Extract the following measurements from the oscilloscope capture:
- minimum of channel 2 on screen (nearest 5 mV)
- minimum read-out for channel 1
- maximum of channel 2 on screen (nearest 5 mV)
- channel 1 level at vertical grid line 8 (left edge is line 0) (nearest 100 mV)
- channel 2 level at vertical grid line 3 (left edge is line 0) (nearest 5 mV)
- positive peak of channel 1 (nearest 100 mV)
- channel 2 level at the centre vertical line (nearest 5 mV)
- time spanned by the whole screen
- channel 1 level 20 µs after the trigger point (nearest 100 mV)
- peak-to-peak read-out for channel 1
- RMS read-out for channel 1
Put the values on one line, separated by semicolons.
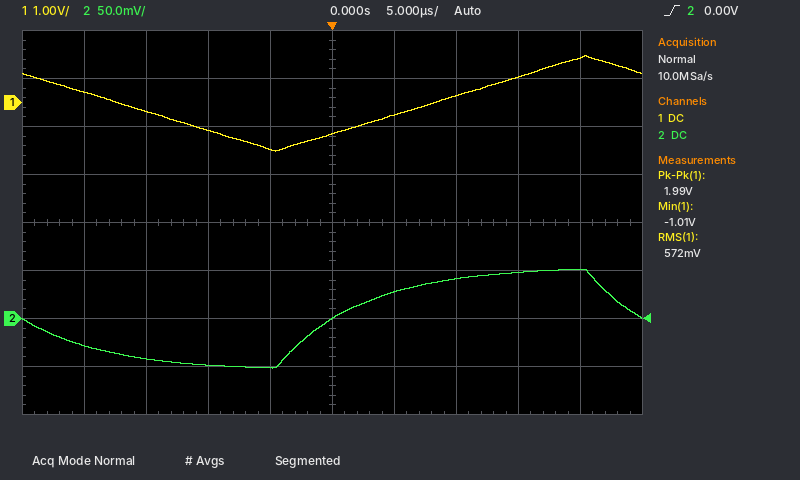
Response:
-50 mV; -1.01 V; 50 mV; 500 mV; -50 mV; 1.0 V; 0 mV; 50 µs; 900 mV; 1.99 V; 572 mV
